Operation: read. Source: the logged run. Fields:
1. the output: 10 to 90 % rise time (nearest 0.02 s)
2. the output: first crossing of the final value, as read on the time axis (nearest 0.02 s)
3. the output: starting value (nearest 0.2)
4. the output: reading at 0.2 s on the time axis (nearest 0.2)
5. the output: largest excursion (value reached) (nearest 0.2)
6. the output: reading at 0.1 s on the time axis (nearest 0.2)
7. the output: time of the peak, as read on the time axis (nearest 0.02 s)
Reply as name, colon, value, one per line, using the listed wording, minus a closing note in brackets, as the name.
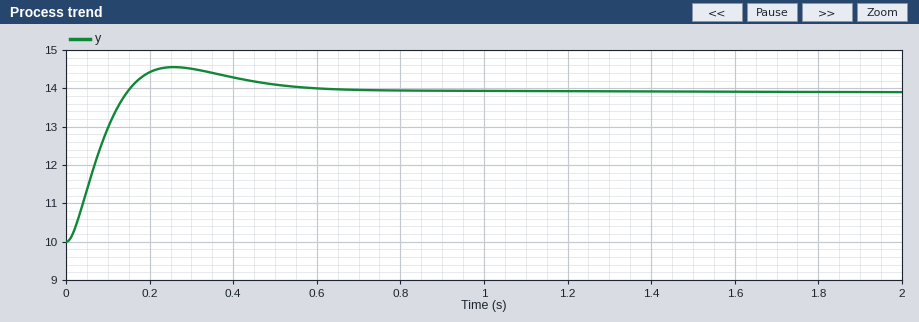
the output: 10 to 90 % rise time: 0.10 s
the output: first crossing of the final value, as read on the time axis: 0.14 s
the output: starting value: 10.0
the output: reading at 0.2 s on the time axis: 14.4
the output: largest excursion (value reached): 14.6
the output: reading at 0.1 s on the time axis: 13.0
the output: time of the peak, as read on the time axis: 0.26 s
